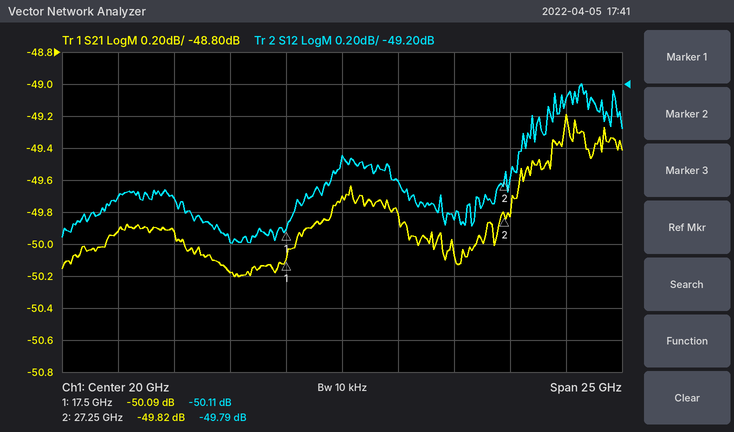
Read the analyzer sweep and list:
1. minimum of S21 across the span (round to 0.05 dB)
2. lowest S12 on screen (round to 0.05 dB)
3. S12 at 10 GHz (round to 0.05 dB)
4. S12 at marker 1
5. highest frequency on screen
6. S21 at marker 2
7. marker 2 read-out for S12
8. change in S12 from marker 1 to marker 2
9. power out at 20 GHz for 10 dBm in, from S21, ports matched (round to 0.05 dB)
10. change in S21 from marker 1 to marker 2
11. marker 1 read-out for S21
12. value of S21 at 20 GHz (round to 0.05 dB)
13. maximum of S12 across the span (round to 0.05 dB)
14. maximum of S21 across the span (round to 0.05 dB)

-50.20 dB
-50.20 dB
-49.90 dB
-50.11 dB
32.5 GHz
-49.82 dB
-49.79 dB
0.32 dB
-39.70 dBm
0.27 dB
-50.09 dB
-49.70 dB
-49.20 dB
-49.20 dB
